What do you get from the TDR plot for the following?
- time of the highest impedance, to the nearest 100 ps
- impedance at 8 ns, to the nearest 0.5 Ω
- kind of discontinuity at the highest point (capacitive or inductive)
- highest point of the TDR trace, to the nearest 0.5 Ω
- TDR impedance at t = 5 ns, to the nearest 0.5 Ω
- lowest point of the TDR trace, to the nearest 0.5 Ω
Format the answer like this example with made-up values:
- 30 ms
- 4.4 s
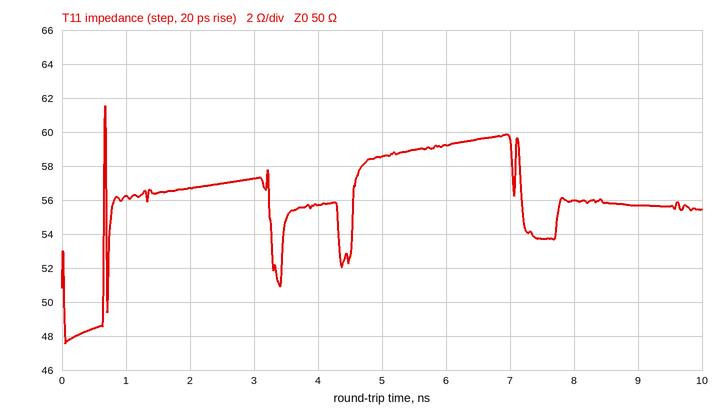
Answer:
- 700 ps
- 56.0 Ω
- inductive
- 61.5 Ω
- 58.5 Ω
- 47.5 Ω
